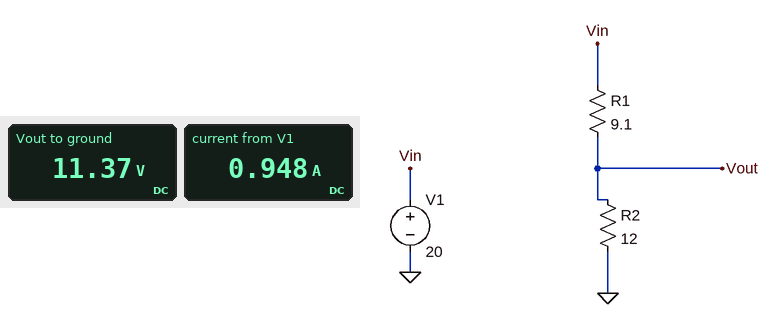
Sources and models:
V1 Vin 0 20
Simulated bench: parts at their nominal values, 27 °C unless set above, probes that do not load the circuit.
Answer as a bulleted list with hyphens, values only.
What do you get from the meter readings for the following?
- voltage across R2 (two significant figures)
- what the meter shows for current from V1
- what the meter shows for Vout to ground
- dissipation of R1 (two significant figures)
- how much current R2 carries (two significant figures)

- 11 V
- 0.948 A
- 11.37 V
- 8.2 W
- 950 mA
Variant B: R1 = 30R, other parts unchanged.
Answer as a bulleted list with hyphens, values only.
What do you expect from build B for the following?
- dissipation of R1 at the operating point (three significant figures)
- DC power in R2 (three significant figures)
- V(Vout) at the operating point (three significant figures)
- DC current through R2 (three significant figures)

- 6.80 W
- 2.72 W
- 5.71 V
- 476 mA
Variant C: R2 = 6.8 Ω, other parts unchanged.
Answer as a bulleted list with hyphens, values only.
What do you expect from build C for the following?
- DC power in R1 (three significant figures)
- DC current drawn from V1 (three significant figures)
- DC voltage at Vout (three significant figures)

- 14.4 W
- 1.26 A
- 8.55 V
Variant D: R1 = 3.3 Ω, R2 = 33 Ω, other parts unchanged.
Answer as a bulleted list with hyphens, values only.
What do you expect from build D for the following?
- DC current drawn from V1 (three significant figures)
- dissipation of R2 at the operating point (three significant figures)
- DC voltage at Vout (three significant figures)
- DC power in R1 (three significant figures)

- 551 mA
- 10.0 W
- 18.2 V
- 1.00 W
